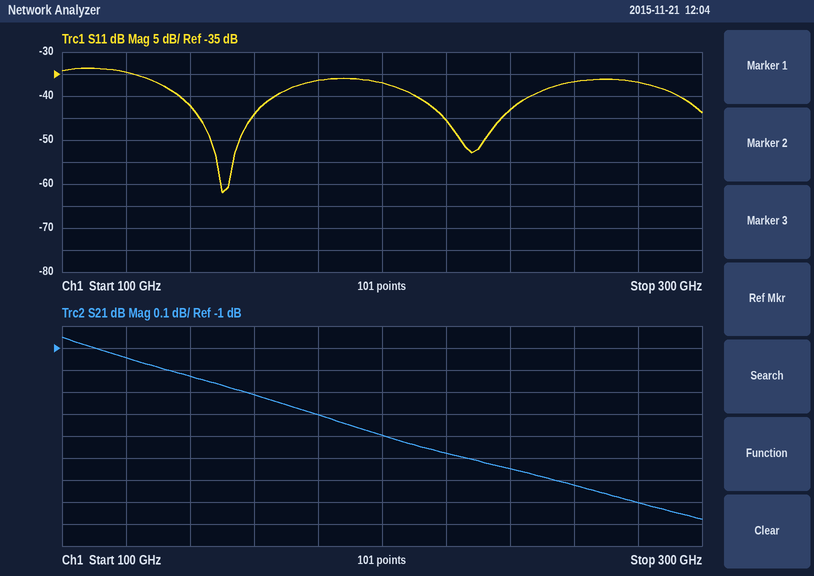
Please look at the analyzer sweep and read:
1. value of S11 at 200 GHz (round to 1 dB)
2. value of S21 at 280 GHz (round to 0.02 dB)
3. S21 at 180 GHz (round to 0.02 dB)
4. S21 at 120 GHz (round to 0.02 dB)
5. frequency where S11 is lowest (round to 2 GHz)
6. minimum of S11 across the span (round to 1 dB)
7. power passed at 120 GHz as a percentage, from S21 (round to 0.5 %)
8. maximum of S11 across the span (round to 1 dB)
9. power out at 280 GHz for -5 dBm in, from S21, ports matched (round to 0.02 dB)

-37 dB
-1.70 dB
-1.30 dB
-1.04 dB
150 GHz
-62 dB
78.5 %
-34 dB
-6.70 dBm
